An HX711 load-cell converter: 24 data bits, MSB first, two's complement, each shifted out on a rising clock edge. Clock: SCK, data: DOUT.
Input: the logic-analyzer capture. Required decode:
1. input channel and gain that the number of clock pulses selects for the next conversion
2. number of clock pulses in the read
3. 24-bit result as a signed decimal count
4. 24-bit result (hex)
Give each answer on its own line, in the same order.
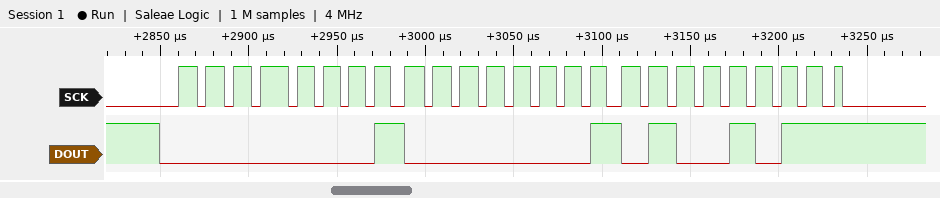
channel A, gain 128
25
65867
0x01014B
